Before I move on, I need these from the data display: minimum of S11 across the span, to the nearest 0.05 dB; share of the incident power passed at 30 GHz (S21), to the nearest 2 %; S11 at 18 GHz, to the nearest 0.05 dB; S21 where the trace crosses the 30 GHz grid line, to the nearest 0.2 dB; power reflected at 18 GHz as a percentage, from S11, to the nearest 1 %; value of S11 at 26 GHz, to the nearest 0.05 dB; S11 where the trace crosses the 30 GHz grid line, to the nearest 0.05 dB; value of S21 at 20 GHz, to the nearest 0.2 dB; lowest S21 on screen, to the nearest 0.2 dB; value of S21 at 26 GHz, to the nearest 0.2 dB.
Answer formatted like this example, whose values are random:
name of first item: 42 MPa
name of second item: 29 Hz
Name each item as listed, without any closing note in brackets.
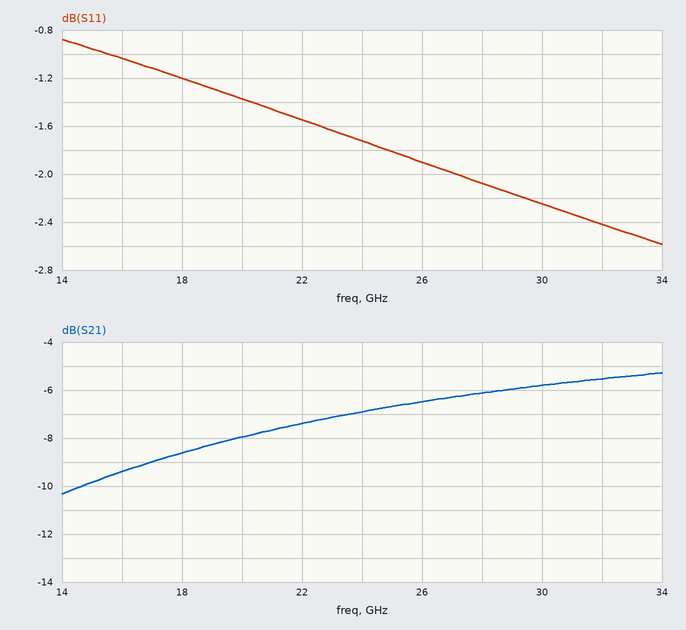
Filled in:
minimum of S11 across the span, to the nearest 0.05 dB: -2.60 dB
share of the incident power passed at 30 GHz (S21), to the nearest 2 %: 26 %
S11 at 18 GHz, to the nearest 0.05 dB: -1.20 dB
S21 where the trace crosses the 30 GHz grid line, to the nearest 0.2 dB: -5.8 dB
power reflected at 18 GHz as a percentage, from S11, to the nearest 1 %: 76 %
value of S11 at 26 GHz, to the nearest 0.05 dB: -1.90 dB
S11 where the trace crosses the 30 GHz grid line, to the nearest 0.05 dB: -2.25 dB
value of S21 at 20 GHz, to the nearest 0.2 dB: -8.0 dB
lowest S21 on screen, to the nearest 0.2 dB: -10.4 dB
value of S21 at 26 GHz, to the nearest 0.2 dB: -6.4 dB
